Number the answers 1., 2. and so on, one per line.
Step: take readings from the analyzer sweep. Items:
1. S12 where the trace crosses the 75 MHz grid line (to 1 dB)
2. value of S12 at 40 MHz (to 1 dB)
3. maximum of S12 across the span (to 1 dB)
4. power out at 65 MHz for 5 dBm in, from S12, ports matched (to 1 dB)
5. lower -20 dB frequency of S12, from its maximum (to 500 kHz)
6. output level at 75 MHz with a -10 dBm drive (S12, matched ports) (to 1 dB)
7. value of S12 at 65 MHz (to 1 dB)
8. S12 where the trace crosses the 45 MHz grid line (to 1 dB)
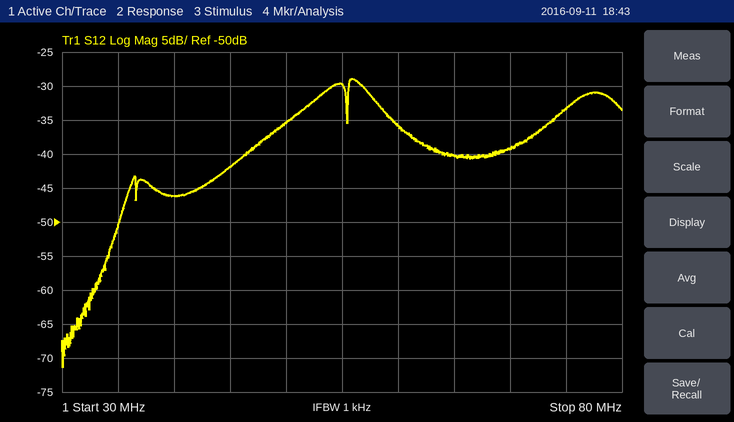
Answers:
1. -33 dB
2. -46 dB
3. -29 dB
4. -35 dBm
5. 35.5 MHz
6. -43 dBm
7. -40 dB
8. -42 dB
